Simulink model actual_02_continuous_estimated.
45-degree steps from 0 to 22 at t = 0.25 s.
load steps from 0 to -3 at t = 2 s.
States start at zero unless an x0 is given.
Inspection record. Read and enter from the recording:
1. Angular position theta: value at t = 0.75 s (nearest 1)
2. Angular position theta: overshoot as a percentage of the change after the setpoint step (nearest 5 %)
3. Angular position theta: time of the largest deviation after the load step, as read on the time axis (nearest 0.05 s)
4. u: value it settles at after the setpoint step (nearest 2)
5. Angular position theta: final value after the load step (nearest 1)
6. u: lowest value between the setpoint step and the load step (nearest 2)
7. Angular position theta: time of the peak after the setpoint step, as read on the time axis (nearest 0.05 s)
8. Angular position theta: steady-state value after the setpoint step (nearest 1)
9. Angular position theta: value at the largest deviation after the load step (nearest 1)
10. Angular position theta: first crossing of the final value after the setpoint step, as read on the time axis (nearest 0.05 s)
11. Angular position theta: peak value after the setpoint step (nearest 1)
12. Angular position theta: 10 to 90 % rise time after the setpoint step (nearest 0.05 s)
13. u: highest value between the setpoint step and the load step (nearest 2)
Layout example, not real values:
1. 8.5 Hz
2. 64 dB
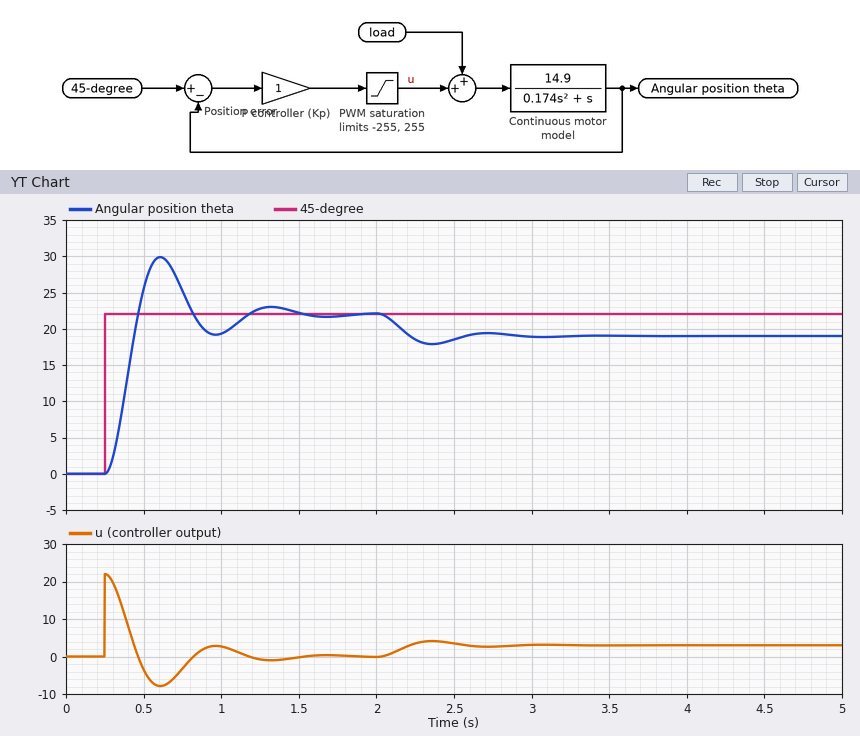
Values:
1. 25
2. 35 %
3. 2.35 s
4. 0
5. 19
6. -8
7. 0.60 s
8. 22
9. 18
10. 0.45 s
11. 30
12. 0.15 s
13. 22
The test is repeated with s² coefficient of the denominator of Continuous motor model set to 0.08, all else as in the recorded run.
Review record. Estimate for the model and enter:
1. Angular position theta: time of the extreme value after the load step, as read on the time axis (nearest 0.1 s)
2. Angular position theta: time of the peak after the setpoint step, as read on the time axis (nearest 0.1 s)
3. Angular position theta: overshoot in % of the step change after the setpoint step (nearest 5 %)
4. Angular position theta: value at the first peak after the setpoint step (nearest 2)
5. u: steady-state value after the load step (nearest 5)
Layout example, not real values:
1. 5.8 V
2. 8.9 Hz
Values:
1. 2.3 s
2. 0.5 s
3. 20 %
4. 26
5. 5
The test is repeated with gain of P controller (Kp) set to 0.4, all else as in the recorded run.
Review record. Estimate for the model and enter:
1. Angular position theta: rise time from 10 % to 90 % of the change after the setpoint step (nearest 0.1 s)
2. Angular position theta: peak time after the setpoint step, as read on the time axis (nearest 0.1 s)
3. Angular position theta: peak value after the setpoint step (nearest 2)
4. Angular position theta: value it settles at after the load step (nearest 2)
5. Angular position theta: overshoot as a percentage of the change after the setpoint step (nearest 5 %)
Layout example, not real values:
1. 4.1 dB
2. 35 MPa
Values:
1. 0.3 s
2. 0.9 s
3. 26
4. 14
5. 15 %
